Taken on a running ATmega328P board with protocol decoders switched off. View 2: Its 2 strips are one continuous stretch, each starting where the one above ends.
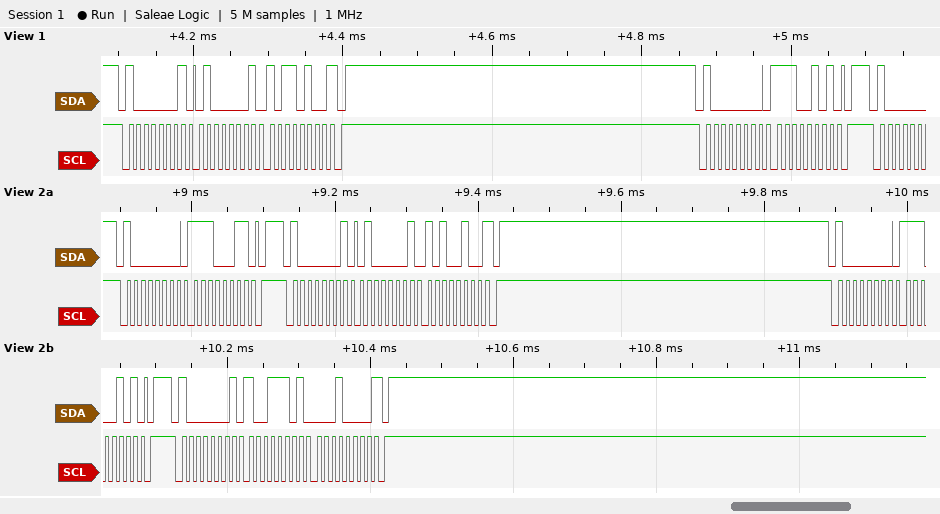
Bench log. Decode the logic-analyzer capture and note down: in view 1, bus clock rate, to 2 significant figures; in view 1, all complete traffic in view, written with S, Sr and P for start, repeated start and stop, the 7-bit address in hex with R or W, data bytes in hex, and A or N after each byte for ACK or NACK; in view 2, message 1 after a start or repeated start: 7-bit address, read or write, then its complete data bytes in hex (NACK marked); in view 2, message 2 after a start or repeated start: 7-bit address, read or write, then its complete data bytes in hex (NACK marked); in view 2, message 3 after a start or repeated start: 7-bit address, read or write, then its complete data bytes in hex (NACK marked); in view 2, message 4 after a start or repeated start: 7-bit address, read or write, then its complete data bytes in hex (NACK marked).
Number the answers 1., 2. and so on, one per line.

1. 100 kHz
2. S 40R A 41 A B4 N P S 40W A E5 A P
3. 0x40 write: E3
4. 0x40 read: 41 A4 NACK
5. 0x40 write: E5
6. 0x40 read: 9D 10 NACK
